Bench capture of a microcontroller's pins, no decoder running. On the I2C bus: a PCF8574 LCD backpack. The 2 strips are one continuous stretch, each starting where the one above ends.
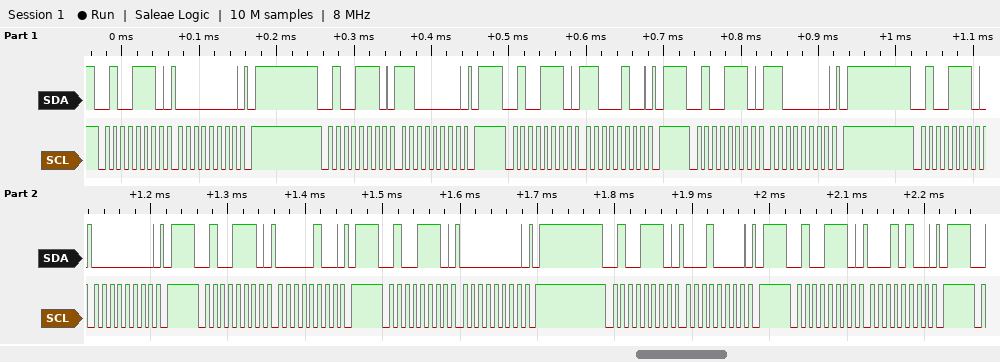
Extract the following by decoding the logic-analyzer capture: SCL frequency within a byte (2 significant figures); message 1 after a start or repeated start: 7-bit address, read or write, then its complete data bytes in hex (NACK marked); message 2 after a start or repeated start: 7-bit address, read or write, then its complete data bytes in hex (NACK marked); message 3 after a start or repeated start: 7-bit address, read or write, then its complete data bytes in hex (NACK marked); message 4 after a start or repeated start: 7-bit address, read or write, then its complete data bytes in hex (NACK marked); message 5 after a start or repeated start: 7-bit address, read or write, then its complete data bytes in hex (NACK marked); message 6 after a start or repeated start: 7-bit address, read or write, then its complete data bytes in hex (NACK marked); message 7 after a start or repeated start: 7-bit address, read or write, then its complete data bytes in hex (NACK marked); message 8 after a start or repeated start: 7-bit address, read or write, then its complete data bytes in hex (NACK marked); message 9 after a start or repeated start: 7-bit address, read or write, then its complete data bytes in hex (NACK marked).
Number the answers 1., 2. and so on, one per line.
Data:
1. 100 kHz
2. 0x27 write: 00
3. 0x27 write: C0
4. 0x27 write: C4
5. 0x27 write: C0
6. 0x27 write: 00
7. 0x27 write: 04
8. 0x27 write: 00
9. 0x27 write: 10
10. 0x27 write: 14
